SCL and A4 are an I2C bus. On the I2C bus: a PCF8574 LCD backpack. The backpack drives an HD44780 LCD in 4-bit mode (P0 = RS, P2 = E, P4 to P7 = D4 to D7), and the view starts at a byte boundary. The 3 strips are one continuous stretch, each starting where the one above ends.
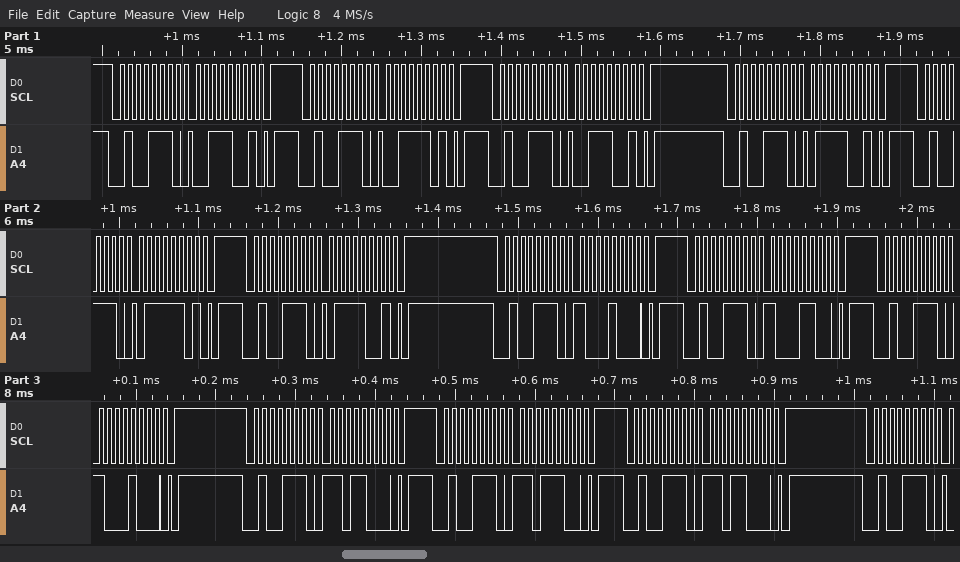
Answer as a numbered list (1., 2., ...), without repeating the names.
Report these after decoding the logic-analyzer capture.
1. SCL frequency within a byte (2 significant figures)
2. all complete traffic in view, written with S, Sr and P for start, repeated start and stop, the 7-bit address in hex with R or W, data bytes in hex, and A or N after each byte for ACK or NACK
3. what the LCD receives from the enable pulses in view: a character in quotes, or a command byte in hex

1. 100 kHz
2. S 27W A 39 A P S 27W A 3D A P S 27W A 39 A P S 27W A 79 A P S 27W A 7D A P S 27W A 79 A P S 27W A 88 A P S 27W A 8C A P S 27W A 88 A P S 27W A D8 A P S 27W A DC A P S 27W A D8 A P S 27W A
3. '7' 0x8D
